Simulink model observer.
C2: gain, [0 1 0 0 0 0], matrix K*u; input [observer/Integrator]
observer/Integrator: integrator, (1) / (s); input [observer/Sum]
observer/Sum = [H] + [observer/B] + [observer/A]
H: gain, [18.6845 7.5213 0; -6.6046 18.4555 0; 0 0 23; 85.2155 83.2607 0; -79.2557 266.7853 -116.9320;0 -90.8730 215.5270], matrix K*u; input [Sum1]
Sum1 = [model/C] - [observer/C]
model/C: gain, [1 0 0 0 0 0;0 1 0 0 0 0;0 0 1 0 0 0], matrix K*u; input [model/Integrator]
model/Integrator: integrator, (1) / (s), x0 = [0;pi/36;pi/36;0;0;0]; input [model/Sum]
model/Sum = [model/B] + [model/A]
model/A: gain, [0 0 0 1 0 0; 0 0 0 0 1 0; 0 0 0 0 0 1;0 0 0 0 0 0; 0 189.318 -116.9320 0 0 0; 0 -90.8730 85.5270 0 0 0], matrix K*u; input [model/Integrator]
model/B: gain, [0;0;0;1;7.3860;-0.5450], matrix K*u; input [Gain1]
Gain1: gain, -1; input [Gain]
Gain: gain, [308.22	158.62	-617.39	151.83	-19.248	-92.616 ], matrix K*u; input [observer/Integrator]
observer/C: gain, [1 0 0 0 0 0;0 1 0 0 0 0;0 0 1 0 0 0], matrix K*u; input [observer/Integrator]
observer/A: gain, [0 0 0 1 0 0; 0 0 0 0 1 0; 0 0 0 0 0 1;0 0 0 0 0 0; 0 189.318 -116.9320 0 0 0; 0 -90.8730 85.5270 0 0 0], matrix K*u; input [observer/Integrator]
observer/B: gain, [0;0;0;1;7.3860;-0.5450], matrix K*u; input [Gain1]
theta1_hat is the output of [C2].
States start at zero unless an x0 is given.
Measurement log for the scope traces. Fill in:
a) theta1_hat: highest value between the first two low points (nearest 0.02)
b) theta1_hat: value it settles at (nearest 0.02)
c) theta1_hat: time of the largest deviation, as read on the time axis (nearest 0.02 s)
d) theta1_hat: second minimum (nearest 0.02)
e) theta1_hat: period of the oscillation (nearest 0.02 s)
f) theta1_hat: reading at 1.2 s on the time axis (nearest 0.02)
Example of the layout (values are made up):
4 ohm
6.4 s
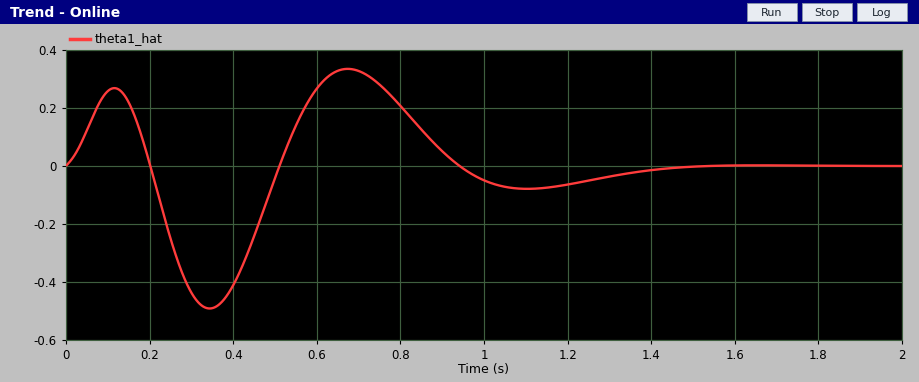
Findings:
0.34
0.00
0.34 s
-0.08
0.76 s
-0.06
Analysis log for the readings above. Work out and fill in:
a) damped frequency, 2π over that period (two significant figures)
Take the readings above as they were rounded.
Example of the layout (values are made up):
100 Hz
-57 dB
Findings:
8.3 rad/s
